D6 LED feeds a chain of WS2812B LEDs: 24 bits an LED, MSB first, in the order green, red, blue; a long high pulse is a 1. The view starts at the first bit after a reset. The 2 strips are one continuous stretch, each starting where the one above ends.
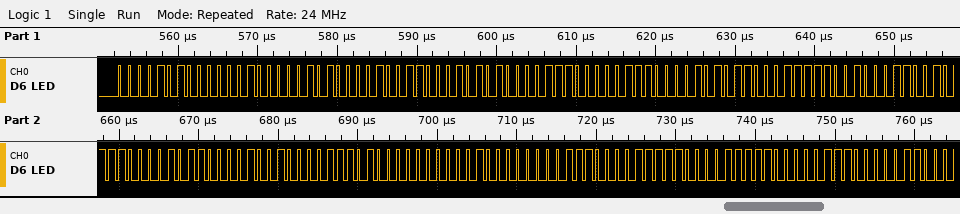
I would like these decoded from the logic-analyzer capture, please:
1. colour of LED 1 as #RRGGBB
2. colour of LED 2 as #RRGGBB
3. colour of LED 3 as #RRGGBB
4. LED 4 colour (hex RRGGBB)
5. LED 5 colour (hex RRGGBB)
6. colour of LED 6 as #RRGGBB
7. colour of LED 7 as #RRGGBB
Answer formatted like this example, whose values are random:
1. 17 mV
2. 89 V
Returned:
1. #040A14
2. #2A261C
3. #2B1C1F
4. #2E2316
5. #1D1200
6. #1C203E
7. #071F06
